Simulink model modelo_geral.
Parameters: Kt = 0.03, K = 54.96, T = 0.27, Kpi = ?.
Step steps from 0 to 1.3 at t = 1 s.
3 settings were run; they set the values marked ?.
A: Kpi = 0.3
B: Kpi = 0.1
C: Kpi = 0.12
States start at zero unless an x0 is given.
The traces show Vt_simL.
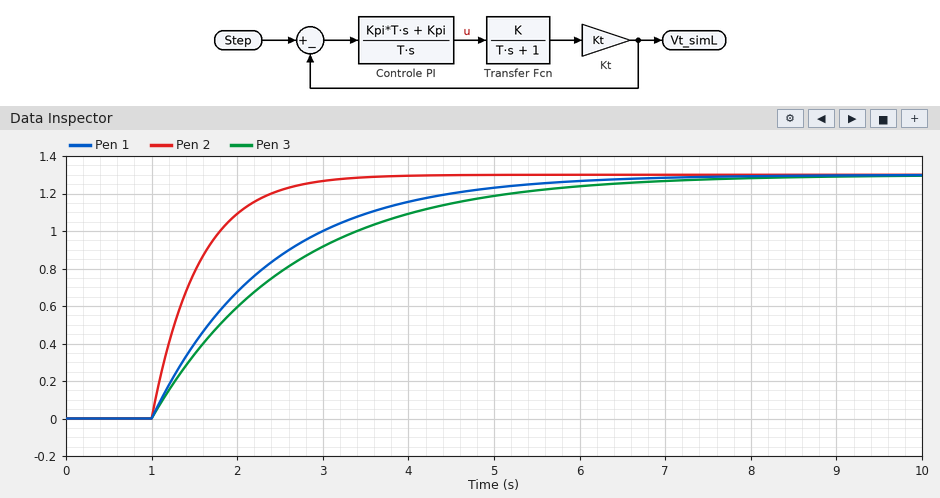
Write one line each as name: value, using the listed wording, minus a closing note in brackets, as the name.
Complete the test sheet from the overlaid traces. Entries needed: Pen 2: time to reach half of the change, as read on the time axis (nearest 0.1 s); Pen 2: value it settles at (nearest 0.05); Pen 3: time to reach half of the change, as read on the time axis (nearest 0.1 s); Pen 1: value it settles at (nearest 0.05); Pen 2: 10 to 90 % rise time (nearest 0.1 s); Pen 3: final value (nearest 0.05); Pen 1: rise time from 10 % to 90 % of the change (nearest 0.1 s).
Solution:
Pen 2: time to reach half of the change, as read on the time axis: 1.4 s
Pen 2: value it settles at: 1.30
Pen 3: time to reach half of the change, as read on the time axis: 2.1 s
Pen 1: value it settles at: 1.30
Pen 2: 10 to 90 % rise time: 1.2 s
Pen 3: final value: 1.30
Pen 1: rise time from 10 % to 90 % of the change: 3.0 s
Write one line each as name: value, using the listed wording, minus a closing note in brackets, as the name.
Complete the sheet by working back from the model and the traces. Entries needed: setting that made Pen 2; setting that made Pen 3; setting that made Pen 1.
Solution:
setting that made Pen 2: A
setting that made Pen 3: B
setting that made Pen 1: C
